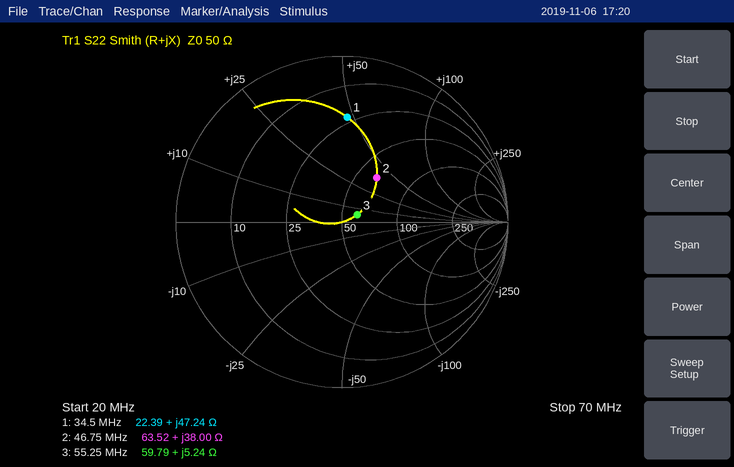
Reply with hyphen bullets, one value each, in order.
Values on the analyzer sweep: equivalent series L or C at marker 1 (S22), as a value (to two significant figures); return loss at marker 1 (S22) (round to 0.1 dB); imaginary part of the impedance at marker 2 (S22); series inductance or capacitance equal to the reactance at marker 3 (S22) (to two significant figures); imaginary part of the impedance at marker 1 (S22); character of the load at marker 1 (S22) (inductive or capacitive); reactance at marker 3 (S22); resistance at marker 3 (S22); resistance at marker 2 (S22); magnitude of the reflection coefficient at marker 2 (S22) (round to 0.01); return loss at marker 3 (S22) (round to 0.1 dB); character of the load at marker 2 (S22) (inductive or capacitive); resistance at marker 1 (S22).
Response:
- 220 nH
- 4.0 dB
- +38.00 Ω
- 15 nH
- +47.24 Ω
- inductive
- +5.24 Ω
- 59.79 Ω
- 63.52 Ω
- 0.34
- 19.9 dB
- inductive
- 22.39 Ω
